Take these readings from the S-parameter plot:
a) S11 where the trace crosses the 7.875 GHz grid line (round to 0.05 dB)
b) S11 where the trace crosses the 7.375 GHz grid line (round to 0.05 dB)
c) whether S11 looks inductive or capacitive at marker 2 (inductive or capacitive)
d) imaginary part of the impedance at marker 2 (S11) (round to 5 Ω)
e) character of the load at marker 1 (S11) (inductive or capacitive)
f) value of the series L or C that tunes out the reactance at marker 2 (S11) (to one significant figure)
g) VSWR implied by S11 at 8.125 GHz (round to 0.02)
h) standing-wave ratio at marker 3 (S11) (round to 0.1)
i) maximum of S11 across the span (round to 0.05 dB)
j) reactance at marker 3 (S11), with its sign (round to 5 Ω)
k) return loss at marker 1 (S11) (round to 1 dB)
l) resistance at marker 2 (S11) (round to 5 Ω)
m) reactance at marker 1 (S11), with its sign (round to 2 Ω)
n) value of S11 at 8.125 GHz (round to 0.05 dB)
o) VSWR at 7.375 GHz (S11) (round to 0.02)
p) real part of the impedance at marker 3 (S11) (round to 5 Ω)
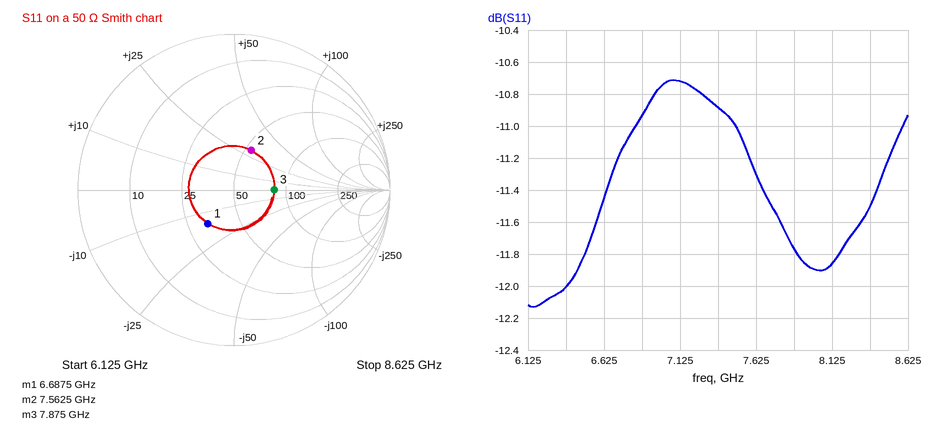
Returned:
-11.75 dB
-10.90 dB
inductive
+30 Ω
capacitive
700 fF
1.68
1.7
-10.70 dB
0 Ω
11 dB
55 Ω
-16 Ω
-11.85 dB
1.80
85 Ω
